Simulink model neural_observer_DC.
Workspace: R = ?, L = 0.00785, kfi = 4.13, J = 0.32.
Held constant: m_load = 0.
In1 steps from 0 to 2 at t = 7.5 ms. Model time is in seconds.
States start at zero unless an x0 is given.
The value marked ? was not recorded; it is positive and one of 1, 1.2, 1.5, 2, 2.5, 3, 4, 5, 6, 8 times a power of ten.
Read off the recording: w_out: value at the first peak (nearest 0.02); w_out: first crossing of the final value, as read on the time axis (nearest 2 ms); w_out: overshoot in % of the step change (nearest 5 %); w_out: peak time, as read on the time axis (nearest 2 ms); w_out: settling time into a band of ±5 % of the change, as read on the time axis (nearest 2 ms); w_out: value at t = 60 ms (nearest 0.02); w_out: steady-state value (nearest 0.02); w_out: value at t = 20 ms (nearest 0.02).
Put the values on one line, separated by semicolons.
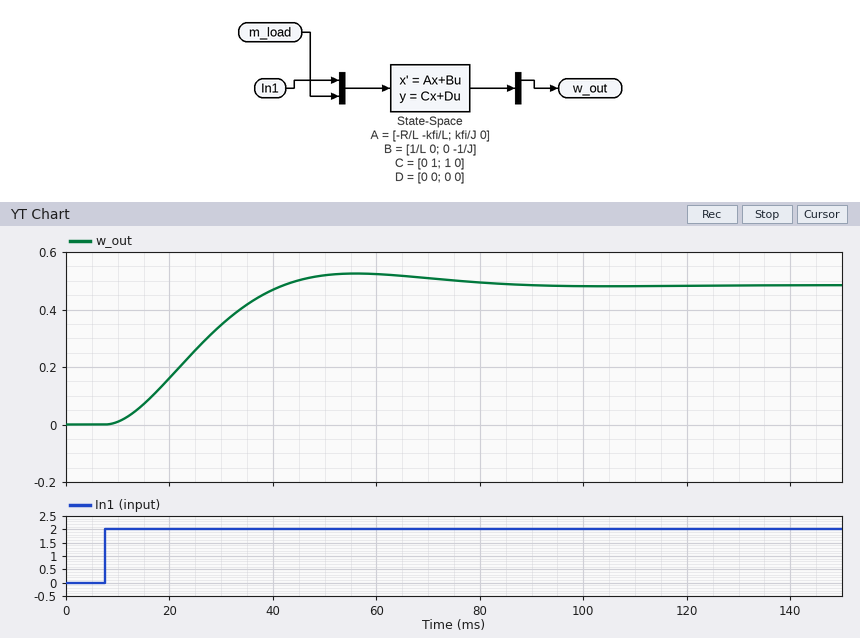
0.52; 42 ms; 10 %; 56 ms; 70 ms; 0.52; 0.48; 0.16
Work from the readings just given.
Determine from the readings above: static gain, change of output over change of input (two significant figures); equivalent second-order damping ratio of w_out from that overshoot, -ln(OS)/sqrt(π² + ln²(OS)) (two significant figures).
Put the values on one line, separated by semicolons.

0.24; 0.59
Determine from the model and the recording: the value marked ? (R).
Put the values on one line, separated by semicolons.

0.8
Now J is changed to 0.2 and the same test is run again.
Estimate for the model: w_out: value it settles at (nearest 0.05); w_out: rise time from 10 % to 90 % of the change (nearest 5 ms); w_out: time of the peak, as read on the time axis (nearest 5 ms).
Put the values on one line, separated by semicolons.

0.50; 15 ms; 40 ms
